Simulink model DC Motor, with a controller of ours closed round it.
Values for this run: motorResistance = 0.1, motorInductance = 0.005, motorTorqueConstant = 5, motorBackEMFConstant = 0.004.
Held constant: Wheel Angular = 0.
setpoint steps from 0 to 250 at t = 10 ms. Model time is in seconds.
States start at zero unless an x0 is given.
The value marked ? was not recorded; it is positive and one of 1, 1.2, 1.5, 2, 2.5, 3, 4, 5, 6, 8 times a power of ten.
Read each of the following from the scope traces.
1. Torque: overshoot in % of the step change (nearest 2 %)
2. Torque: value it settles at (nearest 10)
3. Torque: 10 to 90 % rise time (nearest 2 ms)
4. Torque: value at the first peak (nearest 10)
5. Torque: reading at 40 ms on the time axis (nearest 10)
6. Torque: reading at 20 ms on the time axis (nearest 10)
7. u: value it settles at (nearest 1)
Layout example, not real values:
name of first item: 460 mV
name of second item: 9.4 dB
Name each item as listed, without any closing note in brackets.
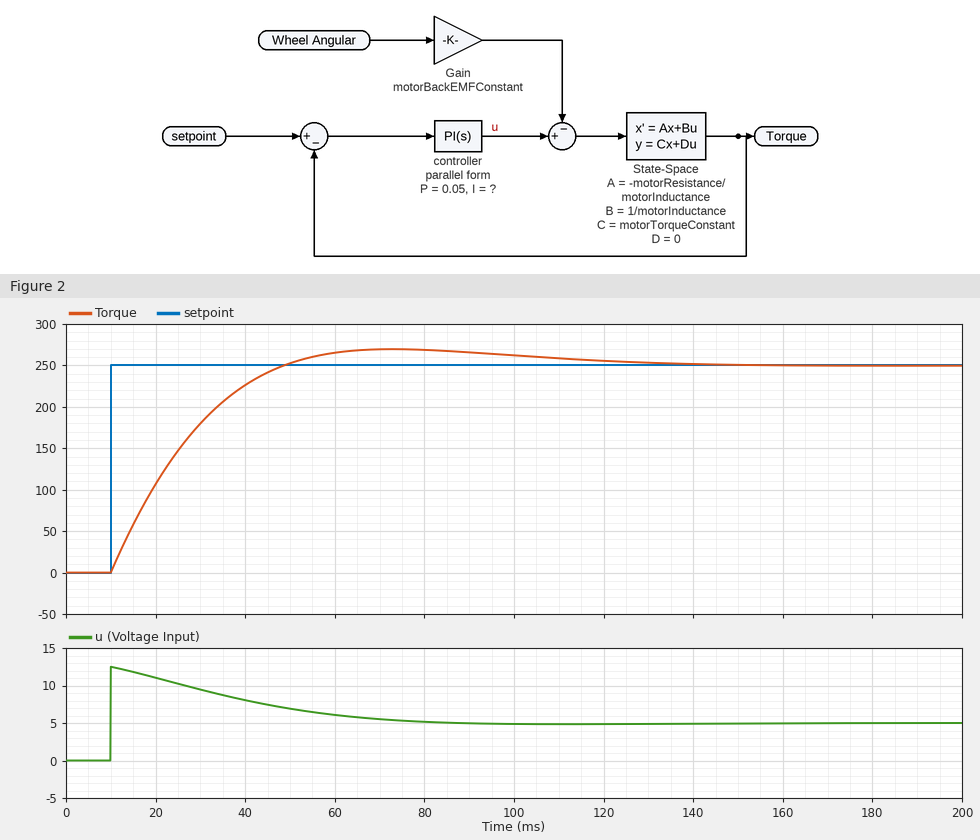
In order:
Torque: overshoot in % of the step change: 8 %
Torque: value it settles at: 250
Torque: 10 to 90 % rise time: 28 ms
Torque: value at the first peak: 270
Torque: reading at 40 ms on the time axis: 230
Torque: reading at 20 ms on the time axis: 110
u: value it settles at: 5
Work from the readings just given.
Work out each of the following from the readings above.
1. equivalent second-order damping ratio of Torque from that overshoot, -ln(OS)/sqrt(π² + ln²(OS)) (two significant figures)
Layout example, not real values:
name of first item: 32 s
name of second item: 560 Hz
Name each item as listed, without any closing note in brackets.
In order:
equivalent second-order damping ratio of Torque from that overshoot, -ln(OS)/sqrt(π² + ln²(OS)): 0.63
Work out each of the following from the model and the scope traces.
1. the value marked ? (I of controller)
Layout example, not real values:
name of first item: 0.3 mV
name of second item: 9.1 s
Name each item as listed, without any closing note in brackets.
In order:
the value marked ?: 2
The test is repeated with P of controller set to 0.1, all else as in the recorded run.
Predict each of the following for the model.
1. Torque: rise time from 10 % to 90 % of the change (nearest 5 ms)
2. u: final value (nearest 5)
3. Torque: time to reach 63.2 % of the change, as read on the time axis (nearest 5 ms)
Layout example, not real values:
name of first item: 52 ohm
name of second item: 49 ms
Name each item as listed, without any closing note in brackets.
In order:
Torque: rise time from 10 % to 90 % of the change: 20 ms
u: final value: 5
Torque: time to reach 63.2 % of the change, as read on the time axis: 20 ms
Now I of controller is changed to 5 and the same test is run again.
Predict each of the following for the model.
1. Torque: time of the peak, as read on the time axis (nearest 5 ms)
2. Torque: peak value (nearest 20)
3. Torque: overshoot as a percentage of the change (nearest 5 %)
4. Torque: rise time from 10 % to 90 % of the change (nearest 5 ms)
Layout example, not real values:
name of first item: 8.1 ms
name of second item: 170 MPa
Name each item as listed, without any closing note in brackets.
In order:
Torque: time of the peak, as read on the time axis: 50 ms
Torque: peak value: 300
Torque: overshoot as a percentage of the change: 25 %
Torque: rise time from 10 % to 90 % of the change: 15 ms
